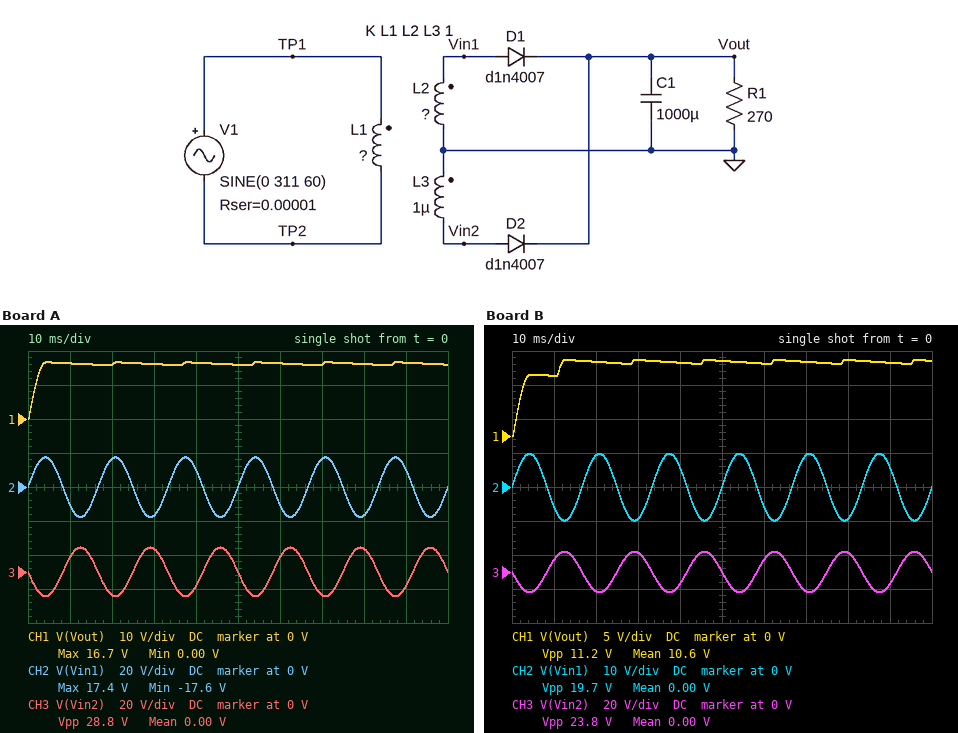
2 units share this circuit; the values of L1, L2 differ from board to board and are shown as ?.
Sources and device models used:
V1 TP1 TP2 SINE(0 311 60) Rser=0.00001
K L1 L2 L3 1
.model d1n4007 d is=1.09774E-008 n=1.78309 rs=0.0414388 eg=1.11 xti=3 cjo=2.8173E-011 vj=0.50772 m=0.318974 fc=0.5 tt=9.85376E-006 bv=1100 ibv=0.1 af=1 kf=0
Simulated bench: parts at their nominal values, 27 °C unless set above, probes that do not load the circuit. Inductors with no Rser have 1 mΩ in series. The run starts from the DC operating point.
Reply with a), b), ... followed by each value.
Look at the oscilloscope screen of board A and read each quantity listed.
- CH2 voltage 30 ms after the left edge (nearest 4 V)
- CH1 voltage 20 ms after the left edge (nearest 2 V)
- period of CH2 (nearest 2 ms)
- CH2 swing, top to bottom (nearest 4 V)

a) -16 V
b) 16 V
c) 16 ms
d) 36 V
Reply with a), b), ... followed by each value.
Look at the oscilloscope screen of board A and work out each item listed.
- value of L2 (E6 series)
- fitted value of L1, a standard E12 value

a) 1.5 µH
b) 470 µH
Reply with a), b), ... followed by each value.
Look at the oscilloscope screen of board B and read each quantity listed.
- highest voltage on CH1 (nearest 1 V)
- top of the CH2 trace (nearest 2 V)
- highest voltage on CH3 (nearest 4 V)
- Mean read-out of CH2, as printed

a) 11 V
b) 10 V
c) 12 V
d) 0.00 V
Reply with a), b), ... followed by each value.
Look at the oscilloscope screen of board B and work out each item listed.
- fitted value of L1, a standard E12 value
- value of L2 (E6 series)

a) 680 µH
b) 680 nH
